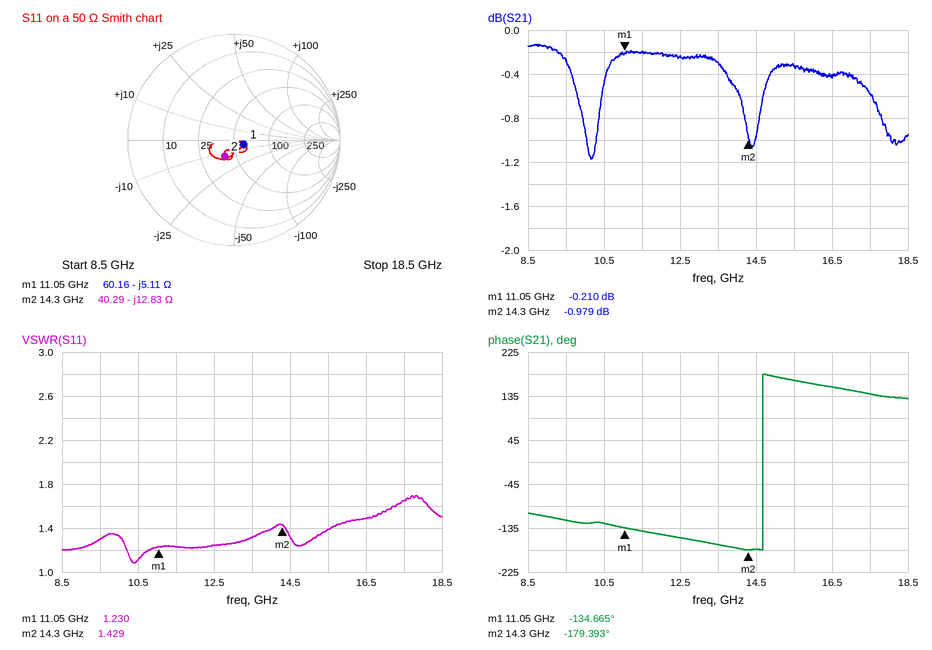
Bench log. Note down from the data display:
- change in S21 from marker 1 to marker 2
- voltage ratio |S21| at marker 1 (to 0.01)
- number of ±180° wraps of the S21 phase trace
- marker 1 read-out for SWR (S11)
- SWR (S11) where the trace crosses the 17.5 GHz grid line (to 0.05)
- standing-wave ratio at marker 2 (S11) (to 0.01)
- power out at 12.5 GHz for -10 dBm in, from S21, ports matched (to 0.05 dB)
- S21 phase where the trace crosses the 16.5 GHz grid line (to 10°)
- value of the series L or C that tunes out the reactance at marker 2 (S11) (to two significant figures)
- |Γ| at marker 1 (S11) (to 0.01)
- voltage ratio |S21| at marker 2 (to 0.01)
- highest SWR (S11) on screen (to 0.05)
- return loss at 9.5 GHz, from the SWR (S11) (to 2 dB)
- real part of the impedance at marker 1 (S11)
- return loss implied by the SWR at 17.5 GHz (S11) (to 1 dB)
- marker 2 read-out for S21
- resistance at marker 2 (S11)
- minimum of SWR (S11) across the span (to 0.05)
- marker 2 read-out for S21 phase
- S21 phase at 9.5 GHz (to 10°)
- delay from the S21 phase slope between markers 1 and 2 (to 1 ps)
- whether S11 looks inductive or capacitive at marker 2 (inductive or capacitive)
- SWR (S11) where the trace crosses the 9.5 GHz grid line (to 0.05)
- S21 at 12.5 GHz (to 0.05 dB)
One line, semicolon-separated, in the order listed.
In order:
-0.769 dB; 0.98; 1; 1.230; 1.65; 1.43; -10.25 dBm; 150°; 140 pH; 0.10; 0.89; 1.70; 18 dB; 60.16 Ω; 12 dB; -0.979 dB; 40.29 Ω; 1.10; -179.393°; -120°; 38 ps; capacitive; 1.30; -0.25 dB
